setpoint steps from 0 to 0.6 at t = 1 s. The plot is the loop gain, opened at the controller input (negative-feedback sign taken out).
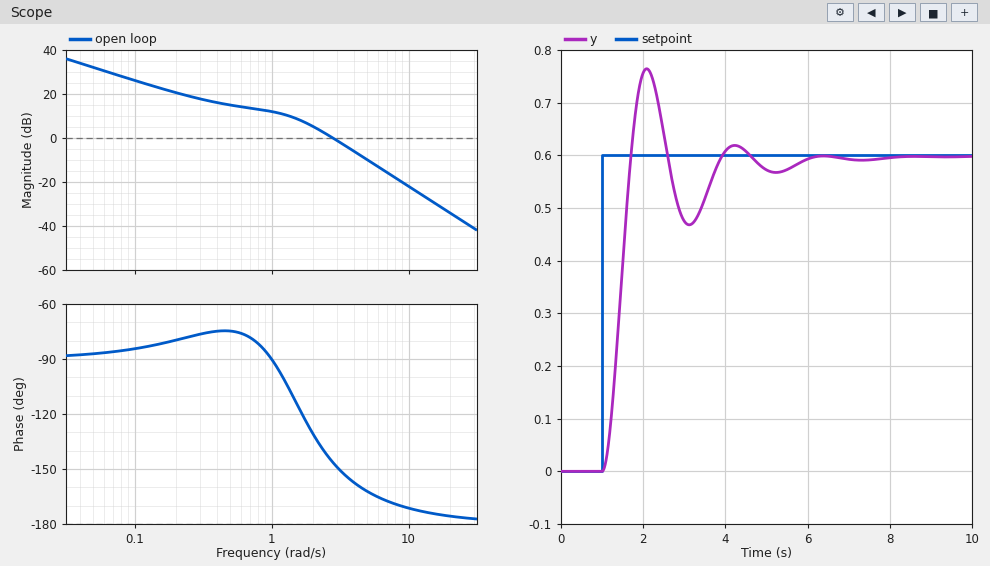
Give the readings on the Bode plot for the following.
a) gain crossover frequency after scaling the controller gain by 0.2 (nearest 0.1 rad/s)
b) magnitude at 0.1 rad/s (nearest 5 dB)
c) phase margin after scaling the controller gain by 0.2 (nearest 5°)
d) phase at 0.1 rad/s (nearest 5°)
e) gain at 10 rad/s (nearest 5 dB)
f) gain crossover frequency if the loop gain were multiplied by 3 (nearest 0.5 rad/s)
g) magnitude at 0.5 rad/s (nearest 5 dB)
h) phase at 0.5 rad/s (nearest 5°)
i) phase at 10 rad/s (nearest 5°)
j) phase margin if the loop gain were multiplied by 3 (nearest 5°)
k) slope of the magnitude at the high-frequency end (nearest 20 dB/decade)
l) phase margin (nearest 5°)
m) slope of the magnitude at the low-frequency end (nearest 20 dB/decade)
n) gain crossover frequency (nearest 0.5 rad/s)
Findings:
0.6 rad/s
25 dB
105°
-85°
-20 dB
5.0 rad/s
15 dB
-75°
-170°
20°
-40 dB/decade
35°
-20 dB/decade
3.0 rad/s
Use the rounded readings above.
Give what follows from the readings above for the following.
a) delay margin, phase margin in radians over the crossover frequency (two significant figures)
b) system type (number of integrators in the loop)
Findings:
0.20 s
1
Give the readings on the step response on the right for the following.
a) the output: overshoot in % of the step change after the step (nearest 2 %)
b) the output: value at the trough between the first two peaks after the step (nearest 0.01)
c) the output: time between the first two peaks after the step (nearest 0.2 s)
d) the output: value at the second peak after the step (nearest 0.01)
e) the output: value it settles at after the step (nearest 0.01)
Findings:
28 %
0.47
2.2 s
0.62
0.60
